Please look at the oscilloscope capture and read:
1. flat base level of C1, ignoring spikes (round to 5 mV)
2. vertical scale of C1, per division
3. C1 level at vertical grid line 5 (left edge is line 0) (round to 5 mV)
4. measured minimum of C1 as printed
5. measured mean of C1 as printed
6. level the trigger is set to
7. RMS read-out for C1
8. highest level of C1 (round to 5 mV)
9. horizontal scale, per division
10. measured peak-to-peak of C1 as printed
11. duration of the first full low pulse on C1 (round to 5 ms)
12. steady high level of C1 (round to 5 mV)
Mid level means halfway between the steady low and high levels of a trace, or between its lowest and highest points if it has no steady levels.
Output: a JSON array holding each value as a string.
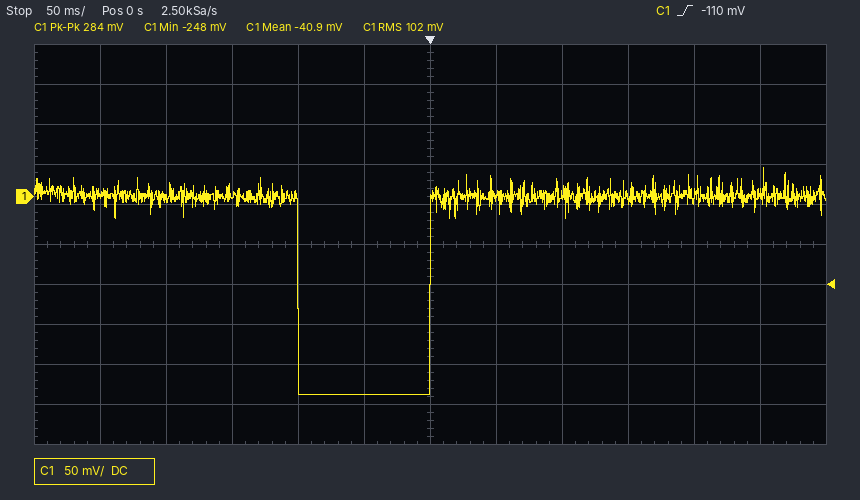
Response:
["-250 mV", "50 mV", "-250 mV", "-248 mV", "-40.9 mV", "-110 mV", "102 mV", "35 mV", "50 ms", "284 mV", "100 ms", "0 mV"]
